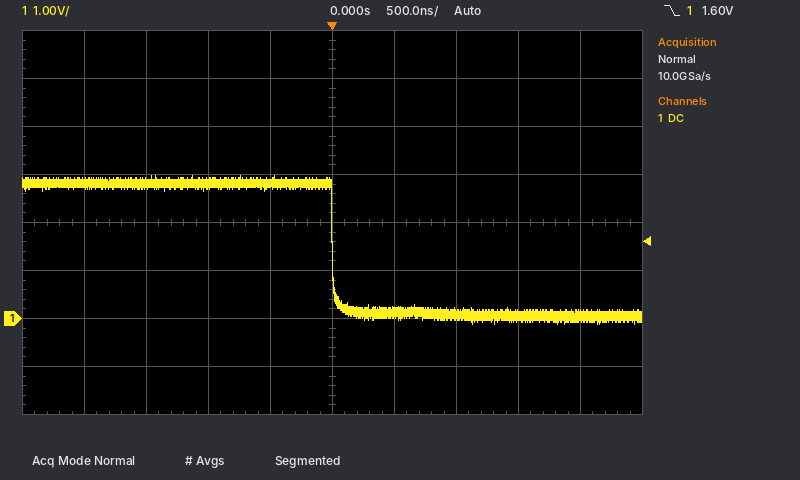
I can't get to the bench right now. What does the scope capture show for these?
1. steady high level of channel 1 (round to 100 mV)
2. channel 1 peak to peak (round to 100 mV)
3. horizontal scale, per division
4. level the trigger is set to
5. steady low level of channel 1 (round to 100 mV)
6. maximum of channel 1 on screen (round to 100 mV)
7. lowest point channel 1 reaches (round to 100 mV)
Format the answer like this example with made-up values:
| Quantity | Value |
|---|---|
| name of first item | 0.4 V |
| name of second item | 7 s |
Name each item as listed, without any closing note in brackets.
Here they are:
| Quantity | Value |
|---|---|
| steady high level of channel 1 | 2.8 V |
| channel 1 peak to peak | 3.1 V |
| horizontal scale, per division | 500 ns |
| level the trigger is set to | 1.60 V |
| steady low level of channel 1 | 100 mV |
| maximum of channel 1 on screen | 3.0 V |
| lowest point channel 1 reaches | -100 mV |
